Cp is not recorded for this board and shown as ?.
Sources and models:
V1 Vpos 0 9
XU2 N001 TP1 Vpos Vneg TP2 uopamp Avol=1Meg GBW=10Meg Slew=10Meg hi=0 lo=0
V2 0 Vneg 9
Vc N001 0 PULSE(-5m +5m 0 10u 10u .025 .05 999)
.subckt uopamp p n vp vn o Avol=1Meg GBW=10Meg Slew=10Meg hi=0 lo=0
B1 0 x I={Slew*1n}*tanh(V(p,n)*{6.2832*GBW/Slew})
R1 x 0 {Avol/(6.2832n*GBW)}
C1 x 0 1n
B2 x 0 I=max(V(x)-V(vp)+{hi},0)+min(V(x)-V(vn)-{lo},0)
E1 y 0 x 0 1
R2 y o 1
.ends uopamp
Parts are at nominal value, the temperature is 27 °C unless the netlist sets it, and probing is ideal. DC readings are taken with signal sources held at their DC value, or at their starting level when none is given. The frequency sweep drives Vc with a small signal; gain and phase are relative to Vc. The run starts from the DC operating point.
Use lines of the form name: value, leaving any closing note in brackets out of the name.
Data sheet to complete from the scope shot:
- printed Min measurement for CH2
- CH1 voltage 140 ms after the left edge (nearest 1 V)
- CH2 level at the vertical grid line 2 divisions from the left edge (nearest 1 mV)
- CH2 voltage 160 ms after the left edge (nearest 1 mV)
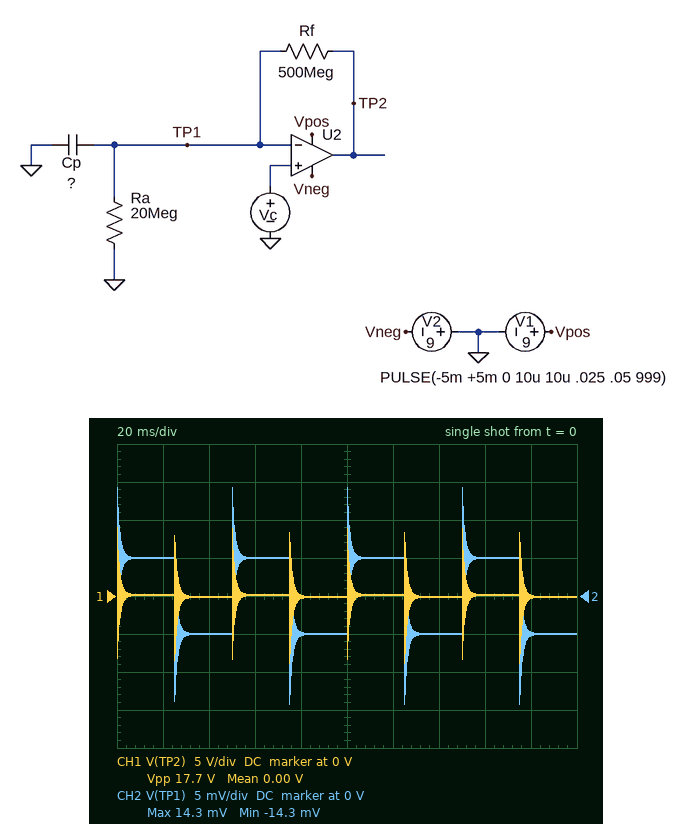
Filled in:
printed Min measurement for CH2: -14.3 mV
CH1 voltage 140 ms after the left edge: 0 V
CH2 level at the vertical grid line 2 divisions from the left edge: -5 mV
CH2 voltage 160 ms after the left edge: 5 mV
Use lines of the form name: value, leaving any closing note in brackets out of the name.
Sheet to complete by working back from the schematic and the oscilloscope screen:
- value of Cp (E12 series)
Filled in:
value of Cp: 27 pF
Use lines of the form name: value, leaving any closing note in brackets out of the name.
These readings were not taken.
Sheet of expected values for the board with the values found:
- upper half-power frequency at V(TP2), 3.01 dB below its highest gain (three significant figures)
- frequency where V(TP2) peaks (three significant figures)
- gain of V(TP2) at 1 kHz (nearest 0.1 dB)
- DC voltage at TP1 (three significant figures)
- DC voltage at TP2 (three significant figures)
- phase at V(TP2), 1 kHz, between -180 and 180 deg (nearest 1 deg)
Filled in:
upper half-power frequency at V(TP2), 3.01 dB below its highest gain: 11.0 kHz
frequency where V(TP2) peaks: 10.9 kHz
gain of V(TP2) at 1 kHz: 39.0 dB
DC voltage at TP1: -5.00 mV
DC voltage at TP2: -130 mV
phase at V(TP2), 1 kHz, between -180 and 180 deg: 73 deg
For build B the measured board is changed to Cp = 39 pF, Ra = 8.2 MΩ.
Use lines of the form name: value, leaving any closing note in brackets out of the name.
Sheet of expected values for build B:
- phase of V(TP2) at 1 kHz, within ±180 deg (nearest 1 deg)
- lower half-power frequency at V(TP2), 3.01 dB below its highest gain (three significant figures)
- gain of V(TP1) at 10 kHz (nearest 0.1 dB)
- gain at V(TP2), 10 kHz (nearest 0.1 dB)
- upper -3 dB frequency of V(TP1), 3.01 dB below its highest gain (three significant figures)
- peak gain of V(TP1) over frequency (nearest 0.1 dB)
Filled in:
phase of V(TP2) at 1 kHz, within ±180 deg: 63 deg
lower half-power frequency at V(TP2), 3.01 dB below its highest gain: 8.78 kHz
gain of V(TP1) at 10 kHz: 12.6 dB
gain at V(TP2), 10 kHz: 74.4 dB
upper -3 dB frequency of V(TP1), 3.01 dB below its highest gain: 9.28 kHz
peak gain of V(TP1) over frequency: 24.9 dB
